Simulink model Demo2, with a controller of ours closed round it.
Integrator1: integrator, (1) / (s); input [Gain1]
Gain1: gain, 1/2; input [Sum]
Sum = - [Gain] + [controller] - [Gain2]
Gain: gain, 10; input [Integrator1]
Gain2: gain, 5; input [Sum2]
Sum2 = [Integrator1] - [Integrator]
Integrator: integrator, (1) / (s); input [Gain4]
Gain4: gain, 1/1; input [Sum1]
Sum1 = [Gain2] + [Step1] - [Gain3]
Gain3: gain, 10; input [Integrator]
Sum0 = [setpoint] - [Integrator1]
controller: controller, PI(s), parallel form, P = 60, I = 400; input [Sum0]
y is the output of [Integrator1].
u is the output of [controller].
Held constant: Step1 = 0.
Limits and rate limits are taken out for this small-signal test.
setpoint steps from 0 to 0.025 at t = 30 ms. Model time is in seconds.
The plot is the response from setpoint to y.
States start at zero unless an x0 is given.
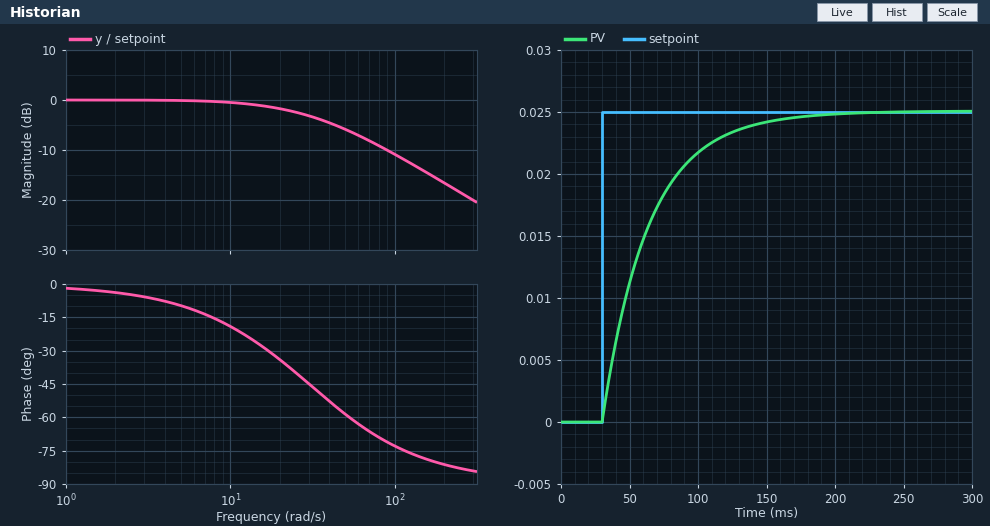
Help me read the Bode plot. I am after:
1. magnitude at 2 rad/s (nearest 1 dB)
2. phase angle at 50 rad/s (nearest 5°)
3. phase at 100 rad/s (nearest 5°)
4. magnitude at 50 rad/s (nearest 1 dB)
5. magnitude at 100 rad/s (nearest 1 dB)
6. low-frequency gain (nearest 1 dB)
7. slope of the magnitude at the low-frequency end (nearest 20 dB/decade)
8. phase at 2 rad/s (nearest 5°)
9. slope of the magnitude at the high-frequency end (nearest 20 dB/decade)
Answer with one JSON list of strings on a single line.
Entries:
["0 dB", "-60°", "-75°", "-6 dB", "-11 dB", "0 dB", "0 dB/decade", "-5°", "-20 dB/decade"]
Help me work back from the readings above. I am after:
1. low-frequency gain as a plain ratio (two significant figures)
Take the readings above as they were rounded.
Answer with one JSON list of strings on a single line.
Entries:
["1.0"]
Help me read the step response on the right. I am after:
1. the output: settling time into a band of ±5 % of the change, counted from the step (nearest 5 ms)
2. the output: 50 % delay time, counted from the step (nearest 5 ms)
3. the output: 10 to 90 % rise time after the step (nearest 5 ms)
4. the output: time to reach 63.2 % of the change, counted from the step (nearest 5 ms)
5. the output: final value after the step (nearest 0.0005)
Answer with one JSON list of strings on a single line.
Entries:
["105 ms", "25 ms", "75 ms", "35 ms", "0.0250"]
